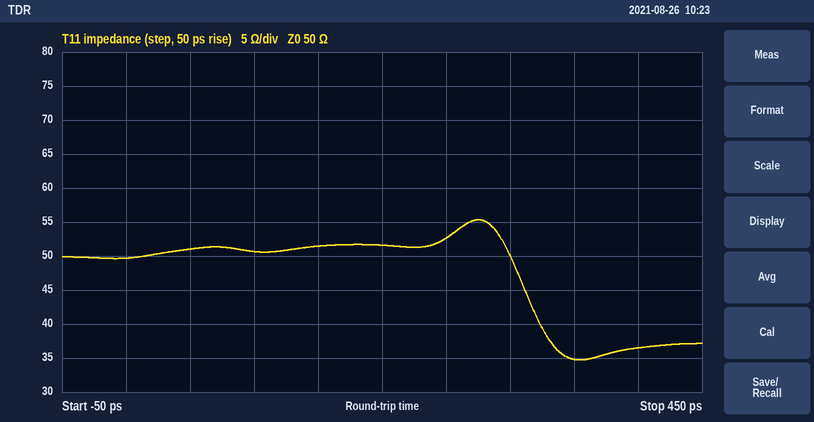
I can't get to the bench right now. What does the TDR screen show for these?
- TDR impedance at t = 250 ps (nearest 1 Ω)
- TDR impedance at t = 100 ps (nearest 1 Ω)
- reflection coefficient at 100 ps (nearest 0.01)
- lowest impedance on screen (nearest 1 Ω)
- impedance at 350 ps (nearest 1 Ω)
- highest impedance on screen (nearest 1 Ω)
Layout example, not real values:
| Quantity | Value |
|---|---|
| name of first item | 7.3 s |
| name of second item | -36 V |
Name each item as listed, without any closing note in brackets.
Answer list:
| Quantity | Value |
|---|---|
| TDR impedance at t = 250 ps | 53 Ω |
| TDR impedance at t = 100 ps | 51 Ω |
| reflection coefficient at 100 ps | +0.01 |
| lowest impedance on screen | 35 Ω |
| impedance at 350 ps | 35 Ω |
| highest impedance on screen | 55 Ω |
